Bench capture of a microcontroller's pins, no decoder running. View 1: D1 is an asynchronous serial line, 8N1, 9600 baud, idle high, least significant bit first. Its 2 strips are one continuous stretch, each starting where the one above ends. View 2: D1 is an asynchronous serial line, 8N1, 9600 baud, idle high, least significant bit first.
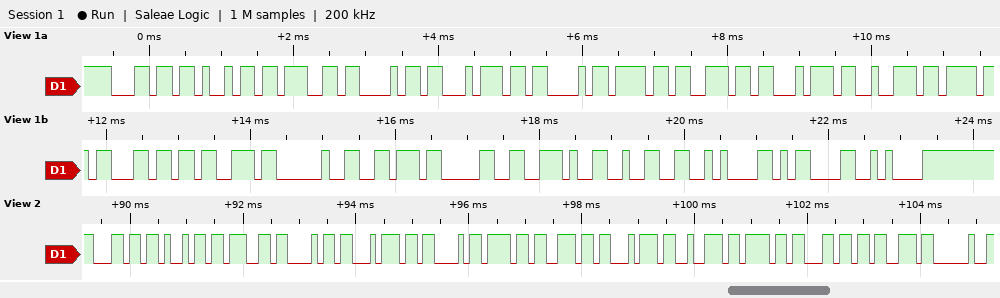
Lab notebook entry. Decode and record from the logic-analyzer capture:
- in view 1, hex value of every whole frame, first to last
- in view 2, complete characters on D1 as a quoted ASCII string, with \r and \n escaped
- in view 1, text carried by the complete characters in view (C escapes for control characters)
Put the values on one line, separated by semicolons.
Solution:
6C 69 67 68 74 43 6F 6E 74 72 6F 6C 73 20 76 30 2E 32 0A 0D 0A; "lightControls "; "lightControls v0.2\n\r\n"
